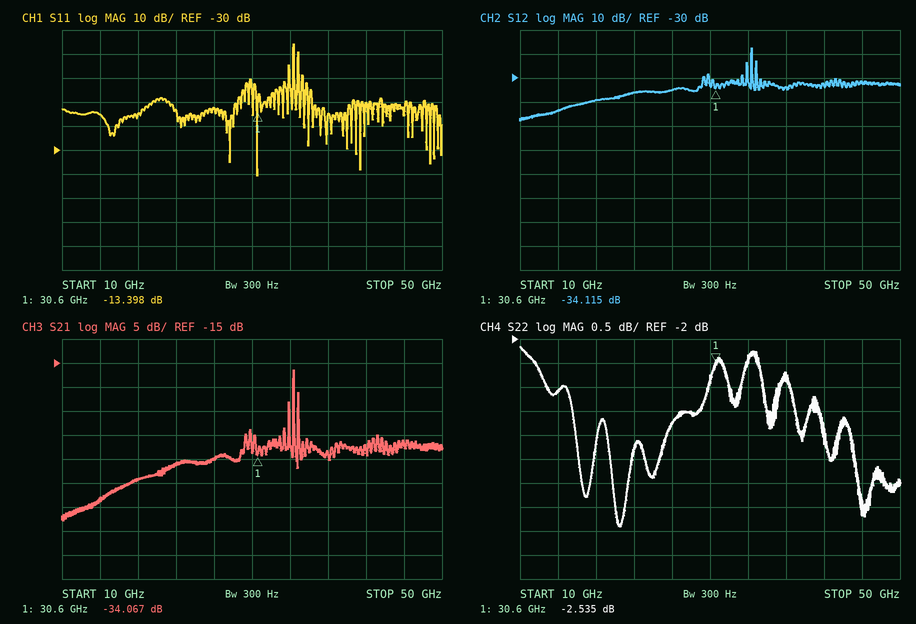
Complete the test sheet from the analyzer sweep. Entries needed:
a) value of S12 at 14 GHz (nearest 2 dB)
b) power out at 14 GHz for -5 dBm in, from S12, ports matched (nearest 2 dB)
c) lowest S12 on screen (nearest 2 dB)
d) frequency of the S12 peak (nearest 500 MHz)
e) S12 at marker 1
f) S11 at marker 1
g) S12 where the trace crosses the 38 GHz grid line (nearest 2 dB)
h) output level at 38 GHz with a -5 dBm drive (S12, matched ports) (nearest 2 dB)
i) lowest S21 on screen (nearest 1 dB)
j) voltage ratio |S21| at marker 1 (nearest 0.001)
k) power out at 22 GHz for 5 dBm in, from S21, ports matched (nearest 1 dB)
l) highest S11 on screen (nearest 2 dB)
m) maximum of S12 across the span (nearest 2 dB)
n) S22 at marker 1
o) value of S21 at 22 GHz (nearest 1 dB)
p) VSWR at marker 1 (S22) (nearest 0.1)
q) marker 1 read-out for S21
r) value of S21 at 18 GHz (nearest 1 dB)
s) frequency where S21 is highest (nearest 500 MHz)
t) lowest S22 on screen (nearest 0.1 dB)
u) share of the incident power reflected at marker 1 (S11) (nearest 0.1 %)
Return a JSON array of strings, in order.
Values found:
["-44 dB", "-48 dBm", "-48 dB", "34.5 GHz", "-34.115 dB", "-13.398 dB", "-34 dB", "-38 dBm", "-48 dB", "0.020", "-31 dBm", "14 dB", "-18 dB", "-2.535 dB", "-36 dB", "6.9", "-34.067 dB", "-39 dB", "34.5 GHz", "-5.9 dB", "4.6 %"]
